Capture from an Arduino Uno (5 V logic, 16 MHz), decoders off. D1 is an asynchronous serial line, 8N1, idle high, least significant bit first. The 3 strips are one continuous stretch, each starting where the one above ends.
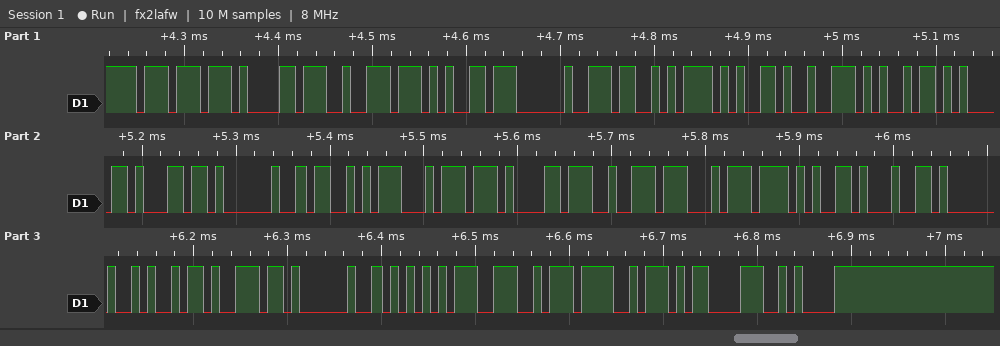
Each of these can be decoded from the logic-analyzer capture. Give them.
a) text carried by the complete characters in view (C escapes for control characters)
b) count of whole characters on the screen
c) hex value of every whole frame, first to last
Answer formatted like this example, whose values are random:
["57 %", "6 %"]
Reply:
["\"ware Serial Started in UNO\\r\\n\"", "28", "77 61 72 65 20 53 65 72 69 61 6C 20 53 74 61 72 74 65 64 20 69 6E 20 55 4E 4F 0D 0A"]
